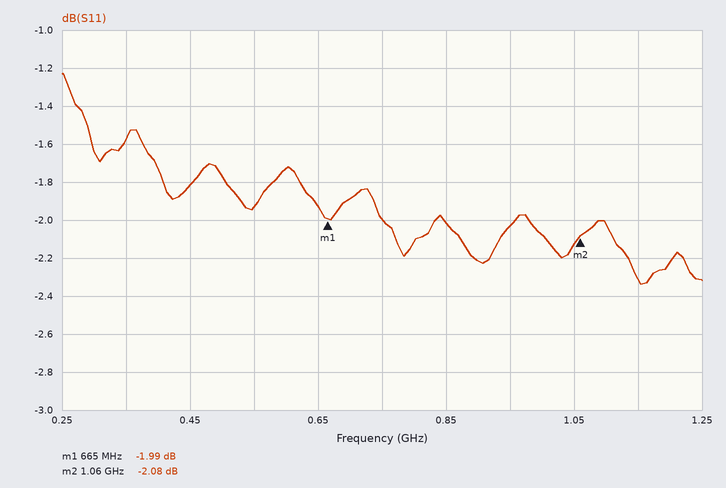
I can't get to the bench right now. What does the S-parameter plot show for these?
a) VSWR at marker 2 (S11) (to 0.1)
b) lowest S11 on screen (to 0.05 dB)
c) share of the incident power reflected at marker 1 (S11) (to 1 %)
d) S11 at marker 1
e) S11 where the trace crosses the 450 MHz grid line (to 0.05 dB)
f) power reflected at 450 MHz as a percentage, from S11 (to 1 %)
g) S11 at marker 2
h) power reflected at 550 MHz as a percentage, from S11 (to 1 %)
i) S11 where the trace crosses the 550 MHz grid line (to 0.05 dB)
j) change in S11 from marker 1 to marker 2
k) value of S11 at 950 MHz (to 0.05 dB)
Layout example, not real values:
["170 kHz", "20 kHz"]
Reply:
["8.4", "-2.35 dB", "63 %", "-1.99 dB", "-1.80 dB", "66 %", "-2.08 dB", "64 %", "-1.95 dB", "-0.09 dB", "-2.05 dB"]
